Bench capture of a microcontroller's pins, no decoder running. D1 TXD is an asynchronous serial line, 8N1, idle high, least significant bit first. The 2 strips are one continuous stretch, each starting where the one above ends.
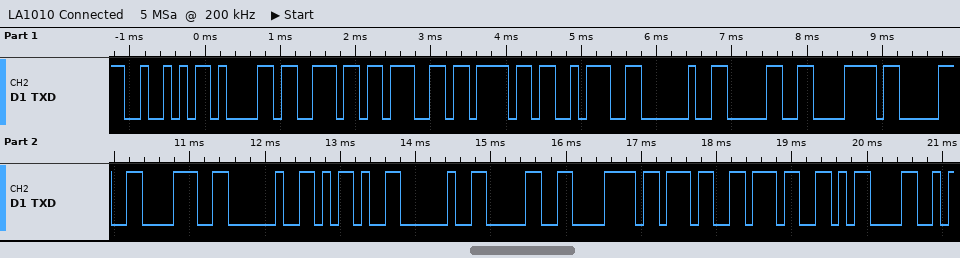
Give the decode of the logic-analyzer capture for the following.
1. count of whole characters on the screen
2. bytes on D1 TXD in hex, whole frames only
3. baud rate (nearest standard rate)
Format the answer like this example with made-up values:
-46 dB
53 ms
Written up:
19
0x52 0x61 0x6E 0x67 0x6F 0x3A 0x20 0x30 0x78 0x30 0x38 0x20 0x2D 0x20 0x30 0x78 0x37 0x37 0x0D
9600 baud
